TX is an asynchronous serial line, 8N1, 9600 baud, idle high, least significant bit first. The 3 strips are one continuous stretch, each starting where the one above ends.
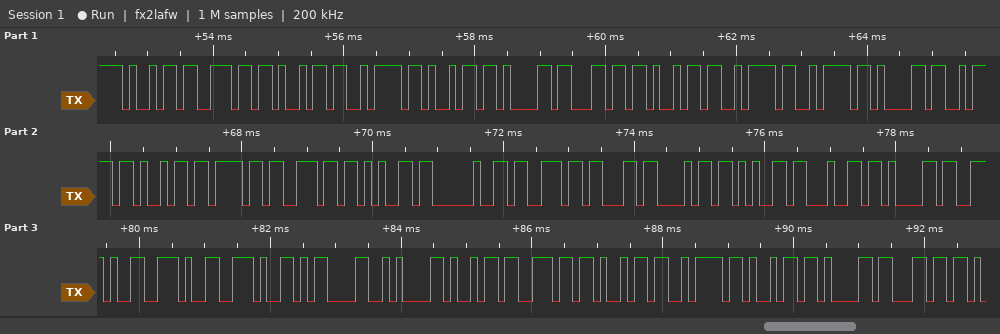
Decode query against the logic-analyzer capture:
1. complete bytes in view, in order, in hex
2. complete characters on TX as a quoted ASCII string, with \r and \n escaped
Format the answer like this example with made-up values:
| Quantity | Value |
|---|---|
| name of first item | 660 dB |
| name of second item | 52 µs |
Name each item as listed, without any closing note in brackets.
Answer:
| Quantity | Value |
|---|---|
| complete bytes in view, in order, in hex | 69 6E 69 7A 69 61 6C 69 7A 7A 61 7A 69 6F 6E 65 20 73 63 68 65 64 61 2E 2E 2E 0D 0A 69 6E 69 7A 69 61 6C |
| complete characters on TX as a quoted ASCII string, with \r and \n escaped | "inizializzazione scheda...\r\ninizial" |
